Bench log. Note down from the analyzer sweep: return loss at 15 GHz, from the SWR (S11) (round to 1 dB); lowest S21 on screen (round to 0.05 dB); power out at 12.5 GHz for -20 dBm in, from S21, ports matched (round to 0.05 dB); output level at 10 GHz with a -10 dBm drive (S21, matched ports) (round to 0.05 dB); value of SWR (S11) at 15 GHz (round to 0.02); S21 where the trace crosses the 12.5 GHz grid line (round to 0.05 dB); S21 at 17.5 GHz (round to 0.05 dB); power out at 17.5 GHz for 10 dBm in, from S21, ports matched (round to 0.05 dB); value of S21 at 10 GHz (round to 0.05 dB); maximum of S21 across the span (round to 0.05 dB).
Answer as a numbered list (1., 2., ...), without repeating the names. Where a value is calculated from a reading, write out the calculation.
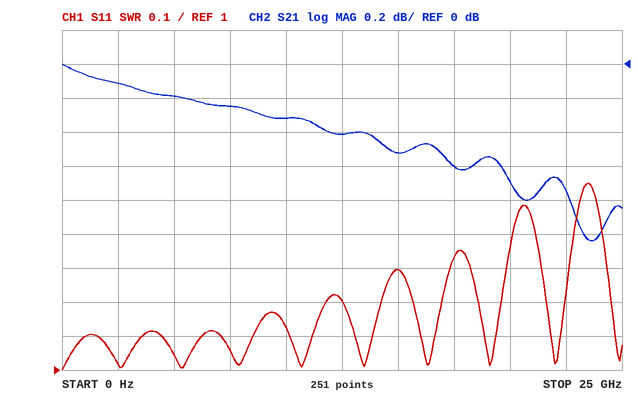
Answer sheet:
1. −20 log10((1.3 − 1)/(1.3 + 1)) ≈ 18 dB
2. -1.05 dB
3. -20 dBm + (-0.40 dB) = -20.40 dBm
4. -10 dBm + (-0.30 dB) = -10.30 dBm
5. 1.30
6. -0.40 dB
7. -0.60 dB
8. 10 dBm + (-0.60 dB) = 9.40 dBm
9. -0.30 dB
10. 0.00 dB
